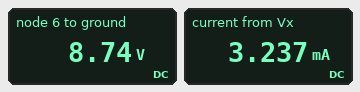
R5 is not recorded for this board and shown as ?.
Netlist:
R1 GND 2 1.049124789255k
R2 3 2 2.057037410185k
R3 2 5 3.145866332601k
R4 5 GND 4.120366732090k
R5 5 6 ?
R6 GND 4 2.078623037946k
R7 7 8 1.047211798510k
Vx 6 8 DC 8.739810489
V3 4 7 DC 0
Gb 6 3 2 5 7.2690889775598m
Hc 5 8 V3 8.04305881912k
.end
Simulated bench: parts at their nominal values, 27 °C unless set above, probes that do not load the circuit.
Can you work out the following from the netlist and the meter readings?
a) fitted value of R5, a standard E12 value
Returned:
2.7 kΩ
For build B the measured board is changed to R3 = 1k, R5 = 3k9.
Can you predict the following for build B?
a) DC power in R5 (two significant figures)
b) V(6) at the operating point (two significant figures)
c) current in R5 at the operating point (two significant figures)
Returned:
20 mW
8.7 V
2.2 mA
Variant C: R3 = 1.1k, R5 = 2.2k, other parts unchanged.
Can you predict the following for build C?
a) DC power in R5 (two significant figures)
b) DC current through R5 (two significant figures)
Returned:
35 mW
4.0 mA
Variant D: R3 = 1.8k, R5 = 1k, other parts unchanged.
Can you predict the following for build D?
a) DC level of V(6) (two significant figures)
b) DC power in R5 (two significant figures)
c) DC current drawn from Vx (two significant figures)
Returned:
8.7 V
76 mW
8.7 mA
